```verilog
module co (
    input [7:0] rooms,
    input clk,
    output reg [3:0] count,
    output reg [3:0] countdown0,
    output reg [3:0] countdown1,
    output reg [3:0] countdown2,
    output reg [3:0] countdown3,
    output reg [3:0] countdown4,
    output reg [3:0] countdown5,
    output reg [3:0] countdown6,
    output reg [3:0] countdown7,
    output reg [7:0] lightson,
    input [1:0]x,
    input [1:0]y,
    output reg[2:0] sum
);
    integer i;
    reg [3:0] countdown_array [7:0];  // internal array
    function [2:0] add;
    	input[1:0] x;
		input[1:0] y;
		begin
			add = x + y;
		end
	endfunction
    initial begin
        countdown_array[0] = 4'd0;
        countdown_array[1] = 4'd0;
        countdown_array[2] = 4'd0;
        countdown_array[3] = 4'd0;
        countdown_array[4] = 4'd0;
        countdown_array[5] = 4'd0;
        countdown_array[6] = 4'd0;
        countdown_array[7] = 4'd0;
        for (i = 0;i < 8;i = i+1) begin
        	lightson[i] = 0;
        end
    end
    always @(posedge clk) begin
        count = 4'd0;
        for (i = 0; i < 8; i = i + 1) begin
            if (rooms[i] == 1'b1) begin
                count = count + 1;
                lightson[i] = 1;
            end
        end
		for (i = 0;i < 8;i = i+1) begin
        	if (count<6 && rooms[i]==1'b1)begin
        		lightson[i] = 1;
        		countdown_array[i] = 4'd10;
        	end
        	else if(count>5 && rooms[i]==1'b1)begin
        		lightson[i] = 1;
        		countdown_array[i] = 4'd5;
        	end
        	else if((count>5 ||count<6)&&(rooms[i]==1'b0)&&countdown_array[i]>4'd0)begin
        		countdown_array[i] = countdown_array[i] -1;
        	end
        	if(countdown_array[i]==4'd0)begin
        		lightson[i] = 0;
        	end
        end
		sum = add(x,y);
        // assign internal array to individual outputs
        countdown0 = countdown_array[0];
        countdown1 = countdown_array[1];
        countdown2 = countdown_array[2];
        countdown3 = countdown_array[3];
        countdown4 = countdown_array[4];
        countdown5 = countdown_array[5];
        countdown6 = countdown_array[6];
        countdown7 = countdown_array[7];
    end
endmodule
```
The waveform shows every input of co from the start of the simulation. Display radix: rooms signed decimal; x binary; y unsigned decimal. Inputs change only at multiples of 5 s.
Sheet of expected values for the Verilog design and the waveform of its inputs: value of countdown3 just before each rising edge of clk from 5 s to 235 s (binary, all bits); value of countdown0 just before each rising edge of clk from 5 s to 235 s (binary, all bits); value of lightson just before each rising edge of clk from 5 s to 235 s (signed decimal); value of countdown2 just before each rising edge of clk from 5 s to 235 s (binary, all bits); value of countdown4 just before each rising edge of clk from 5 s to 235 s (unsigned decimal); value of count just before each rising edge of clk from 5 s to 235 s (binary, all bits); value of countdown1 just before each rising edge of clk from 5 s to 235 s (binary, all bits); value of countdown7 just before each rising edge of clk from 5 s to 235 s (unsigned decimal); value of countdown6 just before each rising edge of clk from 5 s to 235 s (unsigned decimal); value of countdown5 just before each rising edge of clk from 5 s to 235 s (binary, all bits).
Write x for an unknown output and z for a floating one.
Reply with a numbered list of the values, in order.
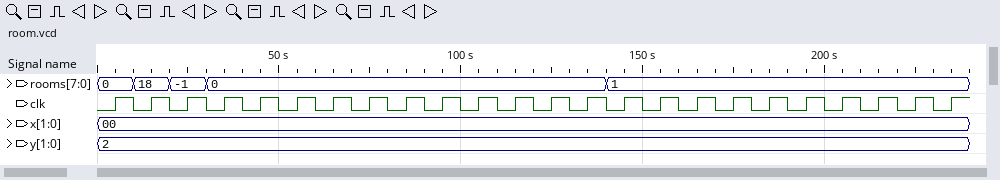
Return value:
1. x, 0000, 0000, 0101, 0100, 0011, 0010, 0001, 0000, 0000, 0000, 0000, 0000, 0000, 0000, 0000, 0000, 0000, 0000, 0000, 0000, 0000, 0000, 0000
2. x, 0000, 0000, 0101, 0100, 0011, 0010, 0001, 0000, 0000, 0000, 0000, 0000, 0000, 0000, 1010, 1010, 1010, 1010, 1010, 1010, 1010, 1010, 1010
3. 0, 0, 18, -1, -1, -1, -1, -1, 0, 0, 0, 0, 0, 0, 0, 1, 1, 1, 1, 1, 1, 1, 1, 1
4. x, 0000, 0000, 0101, 0100, 0011, 0010, 0001, 0000, 0000, 0000, 0000, 0000, 0000, 0000, 0000, 0000, 0000, 0000, 0000, 0000, 0000, 0000, 0000
5. x, 0, 10, 5, 4, 3, 2, 1, 0, 0, 0, 0, 0, 0, 0, 0, 0, 0, 0, 0, 0, 0, 0, 0
6. x, 0000, 0010, 1000, 0000, 0000, 0000, 0000, 0000, 0000, 0000, 0000, 0000, 0000, 0000, 0001, 0001, 0001, 0001, 0001, 0001, 0001, 0001, 0001
7. x, 0000, 1010, 0101, 0100, 0011, 0010, 0001, 0000, 0000, 0000, 0000, 0000, 0000, 0000, 0000, 0000, 0000, 0000, 0000, 0000, 0000, 0000, 0000
8. x, 0, 0, 5, 4, 3, 2, 1, 0, 0, 0, 0, 0, 0, 0, 0, 0, 0, 0, 0, 0, 0, 0, 0
9. x, 0, 0, 5, 4, 3, 2, 1, 0, 0, 0, 0, 0, 0, 0, 0, 0, 0, 0, 0, 0, 0, 0, 0
10. x, 0000, 0000, 0101, 0100, 0011, 0010, 0001, 0000, 0000, 0000, 0000, 0000, 0000, 0000, 0000, 0000, 0000, 0000, 0000, 0000, 0000, 0000, 0000
